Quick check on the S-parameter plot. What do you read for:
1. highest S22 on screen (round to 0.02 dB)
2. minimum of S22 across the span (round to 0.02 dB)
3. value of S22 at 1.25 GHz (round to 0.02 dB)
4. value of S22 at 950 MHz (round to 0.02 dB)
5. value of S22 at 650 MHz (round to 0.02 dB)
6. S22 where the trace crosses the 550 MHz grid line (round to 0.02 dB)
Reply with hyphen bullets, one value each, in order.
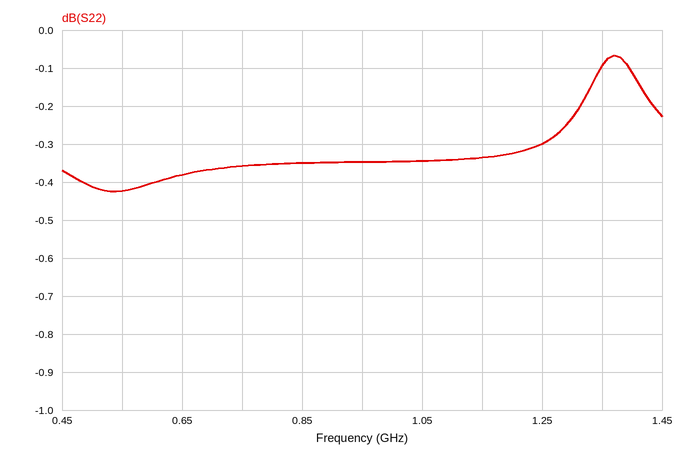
- -0.06 dB
- -0.42 dB
- -0.30 dB
- -0.34 dB
- -0.38 dB
- -0.42 dB
